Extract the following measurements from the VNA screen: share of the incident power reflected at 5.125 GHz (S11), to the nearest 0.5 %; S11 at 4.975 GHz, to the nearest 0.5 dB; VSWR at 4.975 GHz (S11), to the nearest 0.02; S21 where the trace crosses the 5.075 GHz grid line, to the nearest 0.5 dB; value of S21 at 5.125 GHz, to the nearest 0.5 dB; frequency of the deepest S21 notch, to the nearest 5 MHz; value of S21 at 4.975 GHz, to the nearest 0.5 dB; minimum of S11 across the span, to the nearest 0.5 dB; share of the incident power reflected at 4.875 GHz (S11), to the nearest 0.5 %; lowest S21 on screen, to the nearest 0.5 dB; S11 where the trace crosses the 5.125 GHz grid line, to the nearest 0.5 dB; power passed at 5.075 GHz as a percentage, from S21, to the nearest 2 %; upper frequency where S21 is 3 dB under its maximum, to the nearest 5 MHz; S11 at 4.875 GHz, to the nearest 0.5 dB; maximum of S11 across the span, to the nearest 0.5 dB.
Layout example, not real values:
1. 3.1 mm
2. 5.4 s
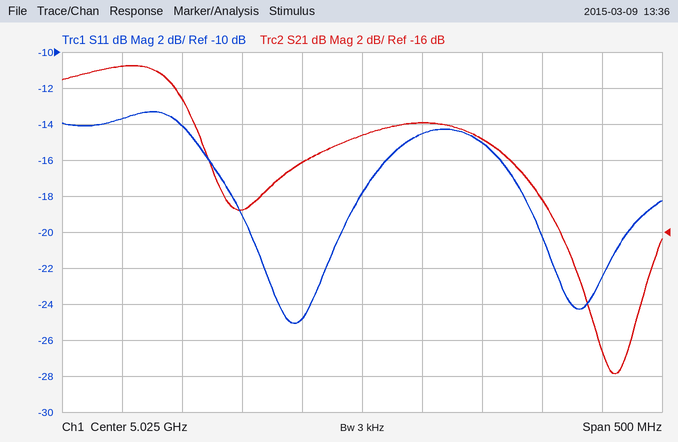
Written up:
1. 3.0 %
2. -25.0 dB
3. 1.12
4. -10.0 dB
5. -11.0 dB
6. 5.235 GHz
7. -12.0 dB
8. -25.0 dB
9. 4.0 %
10. -24.0 dB
11. -15.0 dB
12. 10 %
13. 4.885 GHz
14. -14.0 dB
15. -13.5 dB
